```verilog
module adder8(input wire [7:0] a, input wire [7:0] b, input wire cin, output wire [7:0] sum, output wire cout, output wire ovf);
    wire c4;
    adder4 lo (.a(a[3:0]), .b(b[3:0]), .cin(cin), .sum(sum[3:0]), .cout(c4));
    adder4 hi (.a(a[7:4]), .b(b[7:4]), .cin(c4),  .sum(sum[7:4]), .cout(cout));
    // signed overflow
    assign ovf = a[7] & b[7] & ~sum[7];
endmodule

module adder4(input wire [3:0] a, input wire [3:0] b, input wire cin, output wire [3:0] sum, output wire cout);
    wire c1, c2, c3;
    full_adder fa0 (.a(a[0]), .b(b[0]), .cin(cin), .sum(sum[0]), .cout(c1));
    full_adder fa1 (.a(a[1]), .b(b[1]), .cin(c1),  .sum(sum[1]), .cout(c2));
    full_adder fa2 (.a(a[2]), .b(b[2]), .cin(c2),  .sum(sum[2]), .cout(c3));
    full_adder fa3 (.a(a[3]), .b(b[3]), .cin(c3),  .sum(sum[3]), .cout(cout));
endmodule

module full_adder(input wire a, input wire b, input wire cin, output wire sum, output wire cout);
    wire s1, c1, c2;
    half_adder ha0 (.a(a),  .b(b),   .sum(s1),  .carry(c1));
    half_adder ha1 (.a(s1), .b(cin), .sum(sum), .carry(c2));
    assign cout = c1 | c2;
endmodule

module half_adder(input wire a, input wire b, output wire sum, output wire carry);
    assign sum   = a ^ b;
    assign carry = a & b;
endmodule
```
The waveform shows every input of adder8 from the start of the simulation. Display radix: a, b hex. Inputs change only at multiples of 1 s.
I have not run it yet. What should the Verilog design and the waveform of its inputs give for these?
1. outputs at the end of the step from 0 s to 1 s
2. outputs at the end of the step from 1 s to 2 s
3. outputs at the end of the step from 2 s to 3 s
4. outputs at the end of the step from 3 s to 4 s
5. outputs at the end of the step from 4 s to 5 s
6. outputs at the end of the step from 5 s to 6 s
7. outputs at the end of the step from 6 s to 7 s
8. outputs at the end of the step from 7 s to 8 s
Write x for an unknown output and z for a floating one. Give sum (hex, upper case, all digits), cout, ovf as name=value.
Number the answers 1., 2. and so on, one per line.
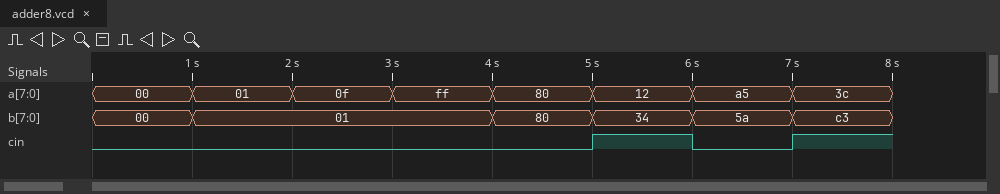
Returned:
1. sum=00, cout=0, ovf=0
2. sum=02, cout=0, ovf=0
3. sum=10, cout=0, ovf=0
4. sum=00, cout=1, ovf=0
5. sum=00, cout=1, ovf=1
6. sum=47, cout=0, ovf=0
7. sum=FF, cout=0, ovf=0
8. sum=00, cout=1, ovf=0
